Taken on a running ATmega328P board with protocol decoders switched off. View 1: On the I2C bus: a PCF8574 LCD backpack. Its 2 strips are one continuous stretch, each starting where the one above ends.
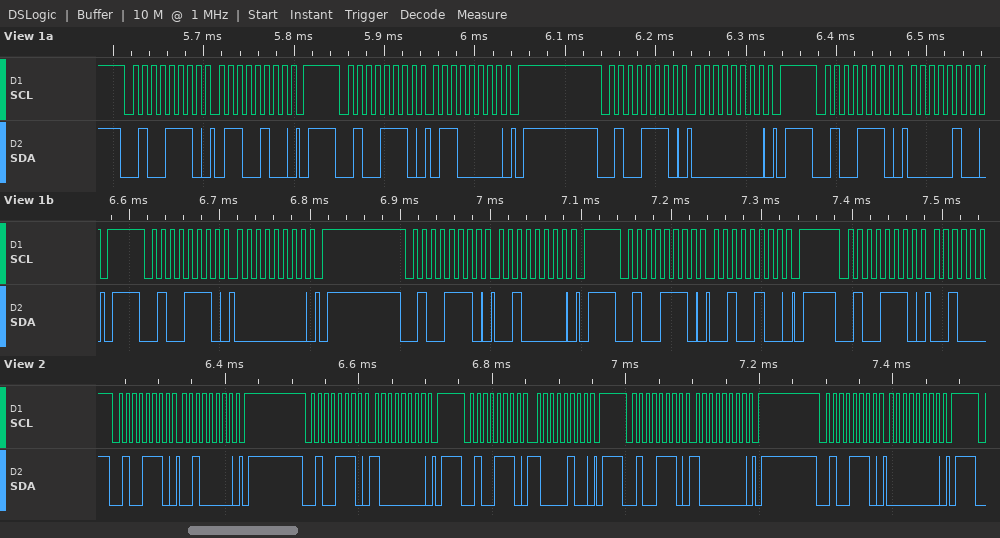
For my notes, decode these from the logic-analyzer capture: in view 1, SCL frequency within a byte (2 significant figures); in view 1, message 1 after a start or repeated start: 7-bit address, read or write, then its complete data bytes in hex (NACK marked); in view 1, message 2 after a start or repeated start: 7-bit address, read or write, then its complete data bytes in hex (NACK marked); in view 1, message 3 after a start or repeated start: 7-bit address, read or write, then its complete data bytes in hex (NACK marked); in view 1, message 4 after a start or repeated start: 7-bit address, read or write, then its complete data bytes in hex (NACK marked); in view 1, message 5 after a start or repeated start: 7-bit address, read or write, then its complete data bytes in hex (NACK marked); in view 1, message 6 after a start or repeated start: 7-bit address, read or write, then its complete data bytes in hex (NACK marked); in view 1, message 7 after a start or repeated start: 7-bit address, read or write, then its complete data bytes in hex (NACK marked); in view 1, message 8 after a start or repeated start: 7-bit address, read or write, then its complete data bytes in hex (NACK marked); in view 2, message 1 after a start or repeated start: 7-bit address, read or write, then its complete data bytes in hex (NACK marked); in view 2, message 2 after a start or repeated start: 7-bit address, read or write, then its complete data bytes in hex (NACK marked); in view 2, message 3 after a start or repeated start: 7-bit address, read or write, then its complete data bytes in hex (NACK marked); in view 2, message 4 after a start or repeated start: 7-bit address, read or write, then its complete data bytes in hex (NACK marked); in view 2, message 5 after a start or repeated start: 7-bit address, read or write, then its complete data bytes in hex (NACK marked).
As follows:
100 kHz
0x27 write: 64
0x27 write: 60
0x27 write: 00
0x27 write: 04
0x27 write: 00
0x27 write: 20
0x27 write: 24
0x27 write
0x27 write: 20
0x27 write: 80
0x27 write: 84
0x27 write: 80
0x27 write: 00
